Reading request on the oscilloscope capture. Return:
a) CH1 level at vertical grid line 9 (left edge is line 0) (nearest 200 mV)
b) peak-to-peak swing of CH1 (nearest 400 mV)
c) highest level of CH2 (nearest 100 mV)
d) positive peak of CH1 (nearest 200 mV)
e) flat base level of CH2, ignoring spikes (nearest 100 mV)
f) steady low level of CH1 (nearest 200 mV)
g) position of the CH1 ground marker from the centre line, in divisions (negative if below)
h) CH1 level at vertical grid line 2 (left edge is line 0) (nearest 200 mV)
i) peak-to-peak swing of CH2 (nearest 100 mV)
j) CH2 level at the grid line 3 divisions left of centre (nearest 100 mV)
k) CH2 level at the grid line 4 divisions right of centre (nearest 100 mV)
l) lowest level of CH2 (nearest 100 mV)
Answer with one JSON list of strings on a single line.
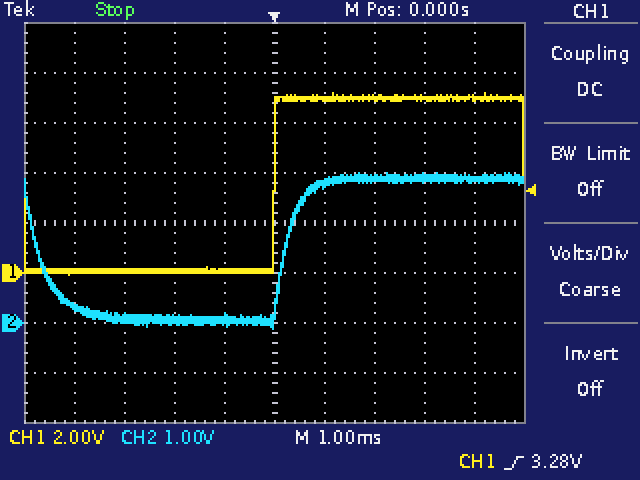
["7.0 V", "7.2 V", "3.0 V", "7.2 V", "100 mV", "0.0 V", "-1.0 div", "0.0 V", "3.1 V", "100 mV", "2.9 V", "-100 mV"]
